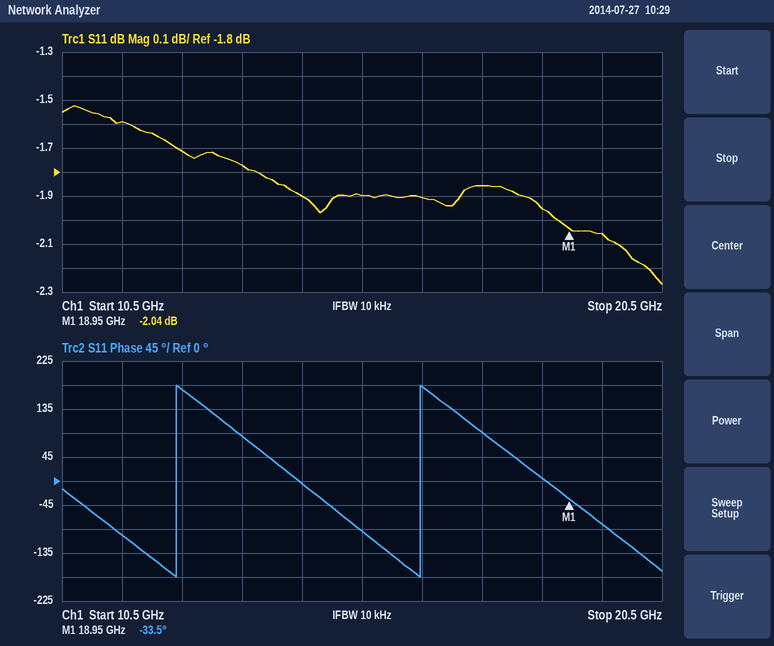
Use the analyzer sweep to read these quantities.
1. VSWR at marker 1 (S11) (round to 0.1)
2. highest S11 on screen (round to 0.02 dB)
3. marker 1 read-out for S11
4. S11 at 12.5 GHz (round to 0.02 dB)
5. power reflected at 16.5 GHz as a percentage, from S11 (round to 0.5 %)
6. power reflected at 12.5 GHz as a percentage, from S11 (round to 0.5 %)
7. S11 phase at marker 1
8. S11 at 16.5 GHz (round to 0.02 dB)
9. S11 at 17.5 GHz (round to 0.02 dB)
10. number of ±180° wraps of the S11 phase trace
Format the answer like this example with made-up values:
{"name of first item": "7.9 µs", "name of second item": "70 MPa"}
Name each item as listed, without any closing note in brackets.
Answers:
{"VSWR at marker 1 (S11)": "8.6", "highest S11 on screen": "-1.52 dB", "marker 1 read-out for S11": "-2.04 dB", "S11 at 12.5 GHz": "-1.72 dB", "power reflected at 16.5 GHz as a percentage, from S11": "64.5 %", "power reflected at 12.5 GHz as a percentage, from S11": "67.5 %", "S11 phase at marker 1": "-33.5°", "S11 at 16.5 GHz": "-1.90 dB", "S11 at 17.5 GHz": "-1.86 dB", "number of ±180° wraps of the S11 phase trace": "2"}
